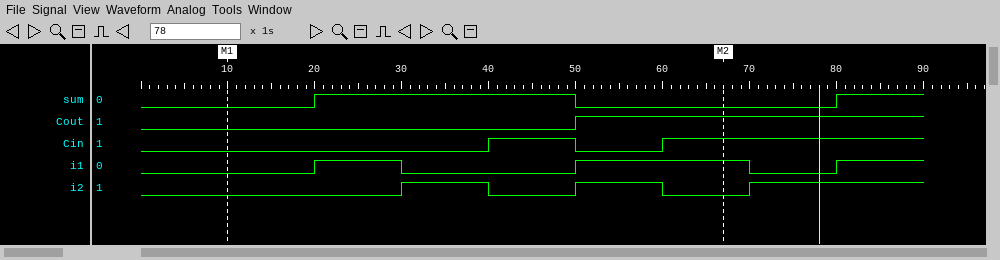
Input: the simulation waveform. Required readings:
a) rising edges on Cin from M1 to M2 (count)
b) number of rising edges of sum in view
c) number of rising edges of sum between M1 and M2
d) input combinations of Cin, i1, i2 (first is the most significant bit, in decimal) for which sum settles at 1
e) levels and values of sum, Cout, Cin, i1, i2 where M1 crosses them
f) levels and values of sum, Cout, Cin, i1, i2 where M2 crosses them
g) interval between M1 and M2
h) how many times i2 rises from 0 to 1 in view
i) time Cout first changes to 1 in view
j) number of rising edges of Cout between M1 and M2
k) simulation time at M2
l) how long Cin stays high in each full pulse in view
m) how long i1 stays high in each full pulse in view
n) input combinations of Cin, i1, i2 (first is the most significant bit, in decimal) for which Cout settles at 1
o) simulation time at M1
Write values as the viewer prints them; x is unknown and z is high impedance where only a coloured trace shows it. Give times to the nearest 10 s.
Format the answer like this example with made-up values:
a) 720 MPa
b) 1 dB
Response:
a) 2
b) 2
c) 1
d) 1, 2, 4, 7
e) sum=0, Cout=0, Cin=0, i1=0, i2=0
f) sum=0, Cout=1, Cin=1, i1=1, i2=0
g) 60 s
h) 3
i) 50 s
j) 1
k) 70 s
l) 10 s
m) 10 s, 20 s
n) 3, 5, 6, 7
o) 10 s
